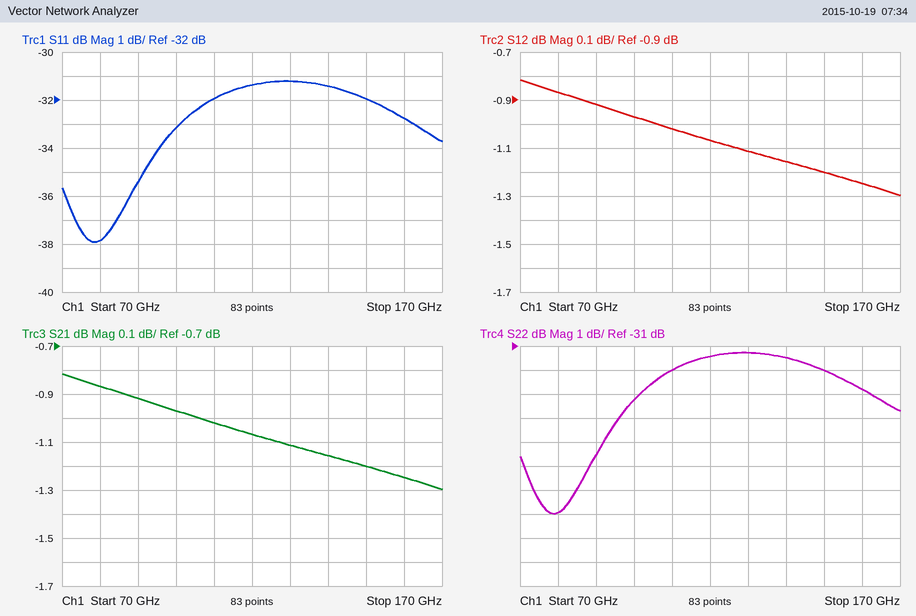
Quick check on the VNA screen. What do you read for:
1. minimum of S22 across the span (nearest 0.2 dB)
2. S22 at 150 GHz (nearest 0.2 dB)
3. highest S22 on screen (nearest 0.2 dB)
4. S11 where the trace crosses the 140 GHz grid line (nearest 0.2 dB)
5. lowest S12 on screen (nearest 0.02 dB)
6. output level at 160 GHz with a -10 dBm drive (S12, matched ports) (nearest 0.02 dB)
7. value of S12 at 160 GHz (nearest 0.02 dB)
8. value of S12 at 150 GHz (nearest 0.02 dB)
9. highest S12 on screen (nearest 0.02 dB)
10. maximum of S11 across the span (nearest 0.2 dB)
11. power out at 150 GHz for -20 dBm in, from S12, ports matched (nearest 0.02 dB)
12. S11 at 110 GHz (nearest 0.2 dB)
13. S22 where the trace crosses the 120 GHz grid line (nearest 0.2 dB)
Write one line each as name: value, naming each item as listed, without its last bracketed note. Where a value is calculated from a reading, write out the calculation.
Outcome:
minimum of S22 across the span: -38.0 dB
S22 at 150 GHz: -32.0 dB
highest S22 on screen: -31.2 dB
S11 where the trace crosses the 140 GHz grid line: -31.4 dB
lowest S12 on screen: -1.30 dB
output level at 160 GHz with a -10 dBm drive (S12, matched ports): -10 dBm + (-1.24 dB) = -11.24 dBm
value of S12 at 160 GHz: -1.24 dB
value of S12 at 150 GHz: -1.20 dB
highest S12 on screen: -0.82 dB
maximum of S11 across the span: -31.2 dB
power out at 150 GHz for -20 dBm in, from S12, ports matched: -20 dBm + (-1.20 dB) = -21.20 dBm
S11 at 110 GHz: -32.0 dB
S22 where the trace crosses the 120 GHz grid line: -31.4 dB
